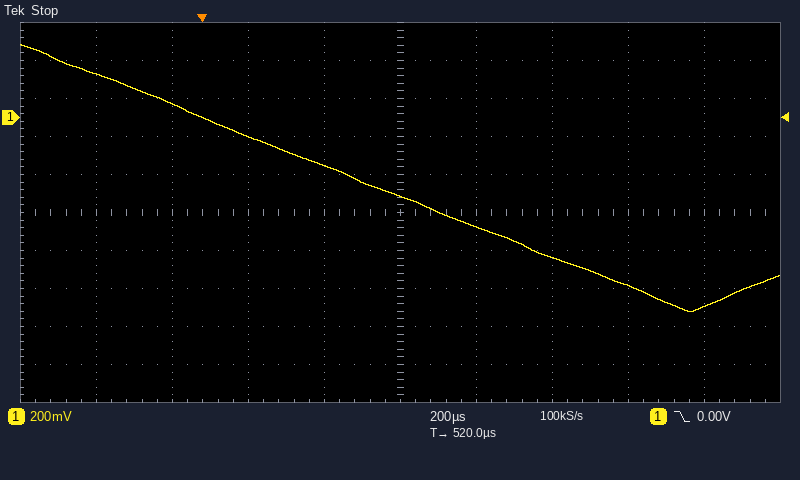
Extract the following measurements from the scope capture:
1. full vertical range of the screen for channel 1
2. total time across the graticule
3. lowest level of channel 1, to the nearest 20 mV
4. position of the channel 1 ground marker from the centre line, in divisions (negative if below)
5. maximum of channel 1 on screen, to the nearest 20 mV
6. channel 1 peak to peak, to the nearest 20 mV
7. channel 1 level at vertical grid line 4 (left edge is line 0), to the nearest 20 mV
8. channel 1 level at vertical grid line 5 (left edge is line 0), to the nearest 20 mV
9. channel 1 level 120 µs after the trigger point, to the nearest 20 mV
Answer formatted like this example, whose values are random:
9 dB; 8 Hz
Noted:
2 V; 2 ms; -1.02 V; +2.5 div; 380 mV; 1.40 V; -260 mV; -420 mV; -100 mV
